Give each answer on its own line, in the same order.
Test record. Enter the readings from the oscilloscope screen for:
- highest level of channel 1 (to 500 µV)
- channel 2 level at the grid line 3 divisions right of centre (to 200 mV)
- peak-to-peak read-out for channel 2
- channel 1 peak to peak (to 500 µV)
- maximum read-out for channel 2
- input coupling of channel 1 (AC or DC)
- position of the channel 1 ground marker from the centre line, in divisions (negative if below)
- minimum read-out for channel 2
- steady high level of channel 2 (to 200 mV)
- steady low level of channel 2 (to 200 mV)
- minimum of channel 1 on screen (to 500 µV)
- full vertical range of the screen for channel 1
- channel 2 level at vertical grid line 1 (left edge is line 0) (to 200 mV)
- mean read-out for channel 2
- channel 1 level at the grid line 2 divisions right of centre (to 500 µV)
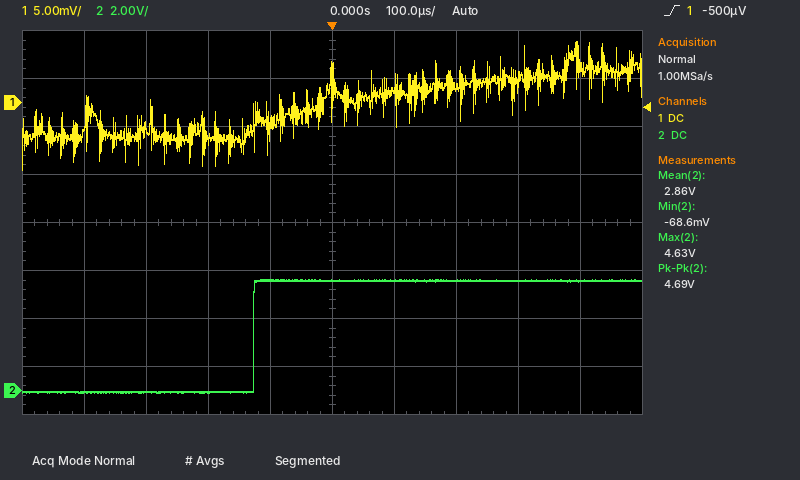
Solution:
6.5 mV
4.6 V
4.69 V
13.5 mV
4.63 V
DC
+2.5 div
-68.6 mV
4.6 V
0.0 V
-7.0 mV
40 mV
0.0 V
2.86 V
1.5 mV
